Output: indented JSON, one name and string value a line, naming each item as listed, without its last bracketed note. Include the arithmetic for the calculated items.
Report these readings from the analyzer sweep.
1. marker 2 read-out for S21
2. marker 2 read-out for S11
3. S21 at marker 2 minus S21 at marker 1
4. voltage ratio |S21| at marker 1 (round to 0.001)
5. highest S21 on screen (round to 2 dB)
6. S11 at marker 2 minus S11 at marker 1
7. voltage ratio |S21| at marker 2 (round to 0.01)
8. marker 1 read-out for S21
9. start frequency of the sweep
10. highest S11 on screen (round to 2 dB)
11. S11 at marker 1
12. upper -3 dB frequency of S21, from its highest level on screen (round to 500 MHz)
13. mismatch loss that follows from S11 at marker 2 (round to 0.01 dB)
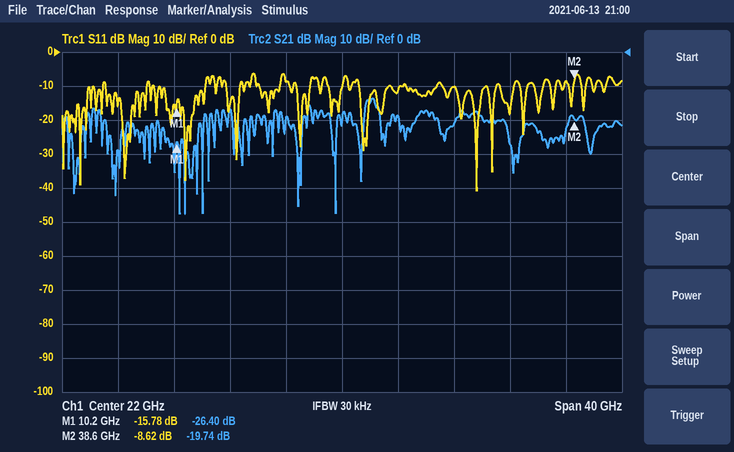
{
  "marker 2 read-out for S21": "-19.74 dB",
  "marker 2 read-out for S11": "-8.62 dB",
  "S21 at marker 2 minus S21 at marker 1": "-19.74 − (-26.4) = 6.66 dB",
  "voltage ratio |S21| at marker 1": "10^(-26.4/20) ≈ 0.048",
  "highest S21 on screen": "-14 dB",
  "S11 at marker 2 minus S11 at marker 1": "-8.62 − (-15.78) = 7.16 dB",
  "voltage ratio |S21| at marker 2": "10^(-19.74/20) ≈ 0.10",
  "marker 1 read-out for S21": "-26.40 dB",
  "start frequency of the sweep": "2 GHz",
  "highest S11 on screen": "-6 dB",
  "S11 at marker 1": "-15.78 dB",
  "upper -3 dB frequency of S21, from its highest level on screen": "24.5 GHz",
  "mismatch loss that follows from S11 at marker 2": "−10 log10(1 − 10^(-8.62/10)) ≈ 0.64 dB"
}
